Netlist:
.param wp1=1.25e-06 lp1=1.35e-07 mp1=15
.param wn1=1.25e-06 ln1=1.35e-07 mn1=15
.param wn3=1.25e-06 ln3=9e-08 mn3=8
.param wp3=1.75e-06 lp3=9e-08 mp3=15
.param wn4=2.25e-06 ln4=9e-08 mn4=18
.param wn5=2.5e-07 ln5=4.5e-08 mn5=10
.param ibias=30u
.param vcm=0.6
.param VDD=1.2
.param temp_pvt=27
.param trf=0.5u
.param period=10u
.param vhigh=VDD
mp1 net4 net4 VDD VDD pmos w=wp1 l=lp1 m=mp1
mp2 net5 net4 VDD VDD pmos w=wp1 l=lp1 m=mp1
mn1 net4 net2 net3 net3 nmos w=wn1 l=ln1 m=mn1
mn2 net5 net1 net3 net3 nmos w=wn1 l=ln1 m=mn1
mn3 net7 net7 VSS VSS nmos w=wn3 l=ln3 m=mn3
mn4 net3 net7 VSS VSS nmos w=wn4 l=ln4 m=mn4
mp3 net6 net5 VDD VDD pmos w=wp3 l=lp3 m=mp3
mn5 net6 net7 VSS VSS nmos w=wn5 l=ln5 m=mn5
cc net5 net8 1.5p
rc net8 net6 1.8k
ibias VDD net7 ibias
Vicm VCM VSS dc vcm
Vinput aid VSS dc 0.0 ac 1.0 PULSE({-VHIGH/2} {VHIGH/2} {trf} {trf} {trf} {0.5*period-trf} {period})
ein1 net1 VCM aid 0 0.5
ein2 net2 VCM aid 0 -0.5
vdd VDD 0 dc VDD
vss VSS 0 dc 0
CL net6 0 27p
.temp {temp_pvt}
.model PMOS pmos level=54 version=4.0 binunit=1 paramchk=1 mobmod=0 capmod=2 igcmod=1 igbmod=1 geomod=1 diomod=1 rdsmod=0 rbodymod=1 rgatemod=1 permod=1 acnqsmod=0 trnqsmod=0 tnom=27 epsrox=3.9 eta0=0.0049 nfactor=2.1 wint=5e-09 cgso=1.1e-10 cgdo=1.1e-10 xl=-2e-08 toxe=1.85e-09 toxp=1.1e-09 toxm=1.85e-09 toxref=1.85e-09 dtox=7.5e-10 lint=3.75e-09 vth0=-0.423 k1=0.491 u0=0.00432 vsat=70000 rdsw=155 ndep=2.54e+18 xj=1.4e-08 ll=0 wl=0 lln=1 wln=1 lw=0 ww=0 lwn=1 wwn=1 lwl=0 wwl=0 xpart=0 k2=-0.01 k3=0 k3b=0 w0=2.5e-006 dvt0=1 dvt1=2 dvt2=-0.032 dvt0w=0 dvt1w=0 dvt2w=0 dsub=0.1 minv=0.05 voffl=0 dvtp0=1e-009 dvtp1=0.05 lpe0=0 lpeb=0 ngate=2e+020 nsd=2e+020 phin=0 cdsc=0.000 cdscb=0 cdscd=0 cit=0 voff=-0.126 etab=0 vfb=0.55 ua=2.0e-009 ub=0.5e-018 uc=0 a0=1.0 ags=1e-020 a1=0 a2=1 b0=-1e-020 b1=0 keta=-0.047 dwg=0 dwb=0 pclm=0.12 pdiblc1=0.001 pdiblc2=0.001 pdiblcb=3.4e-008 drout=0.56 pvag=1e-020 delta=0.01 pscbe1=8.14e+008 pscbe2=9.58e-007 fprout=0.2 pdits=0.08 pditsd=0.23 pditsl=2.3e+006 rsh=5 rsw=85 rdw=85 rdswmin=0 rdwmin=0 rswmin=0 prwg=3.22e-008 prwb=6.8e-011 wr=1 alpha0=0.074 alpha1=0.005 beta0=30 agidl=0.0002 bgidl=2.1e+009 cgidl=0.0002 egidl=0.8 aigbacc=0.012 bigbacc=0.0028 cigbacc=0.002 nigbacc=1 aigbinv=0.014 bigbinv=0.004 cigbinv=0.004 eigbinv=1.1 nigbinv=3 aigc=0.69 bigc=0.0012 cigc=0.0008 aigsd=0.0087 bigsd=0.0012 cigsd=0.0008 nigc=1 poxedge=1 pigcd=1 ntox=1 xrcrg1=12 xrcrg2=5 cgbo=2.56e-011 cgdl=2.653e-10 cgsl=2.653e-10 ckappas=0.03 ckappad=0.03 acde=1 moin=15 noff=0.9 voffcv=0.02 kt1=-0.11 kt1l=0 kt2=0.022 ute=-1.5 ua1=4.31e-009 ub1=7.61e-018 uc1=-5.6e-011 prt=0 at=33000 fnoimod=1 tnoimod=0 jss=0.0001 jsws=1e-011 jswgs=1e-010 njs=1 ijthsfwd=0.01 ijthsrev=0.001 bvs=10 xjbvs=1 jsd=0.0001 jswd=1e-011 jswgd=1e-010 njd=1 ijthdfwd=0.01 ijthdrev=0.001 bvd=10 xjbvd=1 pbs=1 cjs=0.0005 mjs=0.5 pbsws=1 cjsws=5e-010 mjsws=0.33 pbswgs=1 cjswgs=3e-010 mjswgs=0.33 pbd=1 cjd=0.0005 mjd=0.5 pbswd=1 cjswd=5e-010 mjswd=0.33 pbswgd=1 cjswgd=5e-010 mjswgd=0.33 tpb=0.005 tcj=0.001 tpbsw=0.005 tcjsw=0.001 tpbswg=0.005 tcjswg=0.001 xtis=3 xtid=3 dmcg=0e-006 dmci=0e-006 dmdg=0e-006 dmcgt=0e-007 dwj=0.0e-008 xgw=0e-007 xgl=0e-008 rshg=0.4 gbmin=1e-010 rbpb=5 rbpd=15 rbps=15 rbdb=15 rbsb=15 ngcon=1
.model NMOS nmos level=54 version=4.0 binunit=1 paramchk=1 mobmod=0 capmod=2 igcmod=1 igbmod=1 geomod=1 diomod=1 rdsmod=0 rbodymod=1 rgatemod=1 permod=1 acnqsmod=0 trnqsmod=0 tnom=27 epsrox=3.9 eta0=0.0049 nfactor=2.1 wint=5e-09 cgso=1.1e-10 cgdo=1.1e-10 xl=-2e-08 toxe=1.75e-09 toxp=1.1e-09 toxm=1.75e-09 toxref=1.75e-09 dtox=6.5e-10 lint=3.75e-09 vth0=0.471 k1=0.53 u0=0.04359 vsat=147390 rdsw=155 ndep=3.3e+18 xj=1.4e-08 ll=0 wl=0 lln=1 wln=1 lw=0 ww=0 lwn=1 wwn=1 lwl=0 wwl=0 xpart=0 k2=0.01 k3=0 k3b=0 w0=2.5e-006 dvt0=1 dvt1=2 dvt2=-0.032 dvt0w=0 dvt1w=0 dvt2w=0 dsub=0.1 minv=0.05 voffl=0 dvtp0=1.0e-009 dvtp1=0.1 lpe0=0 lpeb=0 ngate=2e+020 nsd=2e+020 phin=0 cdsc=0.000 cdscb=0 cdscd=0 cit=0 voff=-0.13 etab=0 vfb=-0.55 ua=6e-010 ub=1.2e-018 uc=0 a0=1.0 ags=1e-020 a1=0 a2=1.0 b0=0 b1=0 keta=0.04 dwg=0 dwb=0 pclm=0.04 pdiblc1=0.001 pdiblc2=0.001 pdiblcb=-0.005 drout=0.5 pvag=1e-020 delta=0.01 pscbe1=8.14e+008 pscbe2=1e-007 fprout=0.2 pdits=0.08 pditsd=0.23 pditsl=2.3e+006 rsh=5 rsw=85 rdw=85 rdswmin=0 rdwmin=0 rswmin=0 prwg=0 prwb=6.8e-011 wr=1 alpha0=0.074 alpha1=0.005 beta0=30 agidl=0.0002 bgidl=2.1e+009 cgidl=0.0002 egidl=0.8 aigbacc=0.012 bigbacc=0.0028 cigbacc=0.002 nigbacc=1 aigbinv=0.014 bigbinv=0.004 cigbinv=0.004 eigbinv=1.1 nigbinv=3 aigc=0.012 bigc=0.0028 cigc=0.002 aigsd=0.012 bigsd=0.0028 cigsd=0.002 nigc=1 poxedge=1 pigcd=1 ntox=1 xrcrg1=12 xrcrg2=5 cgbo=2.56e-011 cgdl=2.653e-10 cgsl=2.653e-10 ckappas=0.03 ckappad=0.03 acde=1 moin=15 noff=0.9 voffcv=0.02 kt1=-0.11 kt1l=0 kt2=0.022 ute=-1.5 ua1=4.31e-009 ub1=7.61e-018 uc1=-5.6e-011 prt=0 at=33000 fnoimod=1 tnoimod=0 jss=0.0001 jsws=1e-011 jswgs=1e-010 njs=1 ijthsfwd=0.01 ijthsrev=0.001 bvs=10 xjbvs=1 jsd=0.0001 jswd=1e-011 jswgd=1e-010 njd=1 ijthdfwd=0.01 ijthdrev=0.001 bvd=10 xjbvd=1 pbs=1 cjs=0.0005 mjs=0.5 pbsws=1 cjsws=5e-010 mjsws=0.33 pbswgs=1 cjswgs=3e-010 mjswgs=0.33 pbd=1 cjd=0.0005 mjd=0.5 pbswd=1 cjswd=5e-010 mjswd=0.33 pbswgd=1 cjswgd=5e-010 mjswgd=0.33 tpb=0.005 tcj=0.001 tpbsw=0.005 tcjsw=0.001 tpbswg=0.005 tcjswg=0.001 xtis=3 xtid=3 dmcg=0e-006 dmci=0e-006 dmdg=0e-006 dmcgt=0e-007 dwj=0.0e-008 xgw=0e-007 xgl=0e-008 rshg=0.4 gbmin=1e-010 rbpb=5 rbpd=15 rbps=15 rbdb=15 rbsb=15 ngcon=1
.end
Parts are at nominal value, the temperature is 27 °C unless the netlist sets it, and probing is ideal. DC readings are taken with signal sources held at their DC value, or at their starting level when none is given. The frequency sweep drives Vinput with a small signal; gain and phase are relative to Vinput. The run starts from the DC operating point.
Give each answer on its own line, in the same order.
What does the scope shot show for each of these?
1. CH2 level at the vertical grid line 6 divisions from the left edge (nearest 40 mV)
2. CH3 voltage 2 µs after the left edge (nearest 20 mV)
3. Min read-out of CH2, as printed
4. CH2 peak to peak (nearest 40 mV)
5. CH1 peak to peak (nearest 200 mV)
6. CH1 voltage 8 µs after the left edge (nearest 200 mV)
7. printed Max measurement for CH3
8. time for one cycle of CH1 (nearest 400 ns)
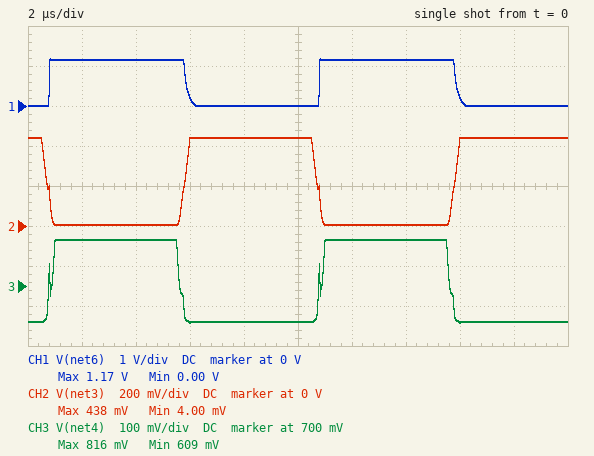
0 V
820 mV
4.00 mV
440 mV
1.2 V
0 V
816 mV
10.0 µs
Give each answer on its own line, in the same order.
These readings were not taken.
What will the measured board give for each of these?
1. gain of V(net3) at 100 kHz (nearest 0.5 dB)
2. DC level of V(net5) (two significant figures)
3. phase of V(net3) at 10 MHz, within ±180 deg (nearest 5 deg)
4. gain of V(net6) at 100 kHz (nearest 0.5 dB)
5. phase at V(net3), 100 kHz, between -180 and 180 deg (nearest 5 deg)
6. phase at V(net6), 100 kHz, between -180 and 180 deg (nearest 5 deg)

-12.5 dB
680 mV
140 deg
49.5 dB
160 deg
-20 deg
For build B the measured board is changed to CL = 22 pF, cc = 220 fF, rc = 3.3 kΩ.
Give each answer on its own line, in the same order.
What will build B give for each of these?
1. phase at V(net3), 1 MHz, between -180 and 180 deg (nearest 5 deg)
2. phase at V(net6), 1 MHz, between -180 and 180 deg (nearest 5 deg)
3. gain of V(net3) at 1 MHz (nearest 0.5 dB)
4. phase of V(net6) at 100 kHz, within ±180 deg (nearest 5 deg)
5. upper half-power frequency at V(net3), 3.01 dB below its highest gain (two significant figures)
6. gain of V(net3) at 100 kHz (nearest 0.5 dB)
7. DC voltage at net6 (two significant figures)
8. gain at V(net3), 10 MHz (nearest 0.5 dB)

155 deg
-45 deg
-14.0 dB
-5 deg
1.4 MHz
-12.0 dB
660 mV
-20.5 dB
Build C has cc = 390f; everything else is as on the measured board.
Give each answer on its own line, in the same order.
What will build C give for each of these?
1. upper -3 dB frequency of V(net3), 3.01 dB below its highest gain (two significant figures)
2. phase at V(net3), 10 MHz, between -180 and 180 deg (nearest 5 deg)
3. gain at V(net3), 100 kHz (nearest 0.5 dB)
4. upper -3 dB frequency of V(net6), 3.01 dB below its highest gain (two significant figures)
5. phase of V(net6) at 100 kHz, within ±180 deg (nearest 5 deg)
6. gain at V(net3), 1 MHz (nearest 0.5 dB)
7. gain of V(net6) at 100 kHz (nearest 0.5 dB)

850 kHz
145 deg
-12.0 dB
750 kHz
-10 deg
-15.5 dB
50.0 dB
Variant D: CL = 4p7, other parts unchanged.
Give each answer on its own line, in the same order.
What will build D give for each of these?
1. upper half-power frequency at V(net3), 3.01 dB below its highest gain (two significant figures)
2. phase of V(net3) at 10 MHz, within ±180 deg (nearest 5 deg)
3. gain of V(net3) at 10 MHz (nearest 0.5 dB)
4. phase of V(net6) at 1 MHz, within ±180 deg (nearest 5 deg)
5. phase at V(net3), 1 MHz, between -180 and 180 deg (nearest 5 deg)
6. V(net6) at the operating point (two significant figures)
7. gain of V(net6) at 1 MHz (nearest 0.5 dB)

280 kHz
130 deg
-41.0 dB
-75 deg
110 deg
660 mV
39.0 dB
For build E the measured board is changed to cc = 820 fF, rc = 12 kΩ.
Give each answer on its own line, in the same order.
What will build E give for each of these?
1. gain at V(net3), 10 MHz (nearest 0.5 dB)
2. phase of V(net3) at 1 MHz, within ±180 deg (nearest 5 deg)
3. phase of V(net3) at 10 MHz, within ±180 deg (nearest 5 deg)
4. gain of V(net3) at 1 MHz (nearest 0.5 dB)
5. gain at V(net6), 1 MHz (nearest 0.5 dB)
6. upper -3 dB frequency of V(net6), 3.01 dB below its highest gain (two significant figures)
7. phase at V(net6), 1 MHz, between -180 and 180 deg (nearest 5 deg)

-27.0 dB
135 deg
165 deg
-19.5 dB
42.0 dB
420 kHz
-70 deg
